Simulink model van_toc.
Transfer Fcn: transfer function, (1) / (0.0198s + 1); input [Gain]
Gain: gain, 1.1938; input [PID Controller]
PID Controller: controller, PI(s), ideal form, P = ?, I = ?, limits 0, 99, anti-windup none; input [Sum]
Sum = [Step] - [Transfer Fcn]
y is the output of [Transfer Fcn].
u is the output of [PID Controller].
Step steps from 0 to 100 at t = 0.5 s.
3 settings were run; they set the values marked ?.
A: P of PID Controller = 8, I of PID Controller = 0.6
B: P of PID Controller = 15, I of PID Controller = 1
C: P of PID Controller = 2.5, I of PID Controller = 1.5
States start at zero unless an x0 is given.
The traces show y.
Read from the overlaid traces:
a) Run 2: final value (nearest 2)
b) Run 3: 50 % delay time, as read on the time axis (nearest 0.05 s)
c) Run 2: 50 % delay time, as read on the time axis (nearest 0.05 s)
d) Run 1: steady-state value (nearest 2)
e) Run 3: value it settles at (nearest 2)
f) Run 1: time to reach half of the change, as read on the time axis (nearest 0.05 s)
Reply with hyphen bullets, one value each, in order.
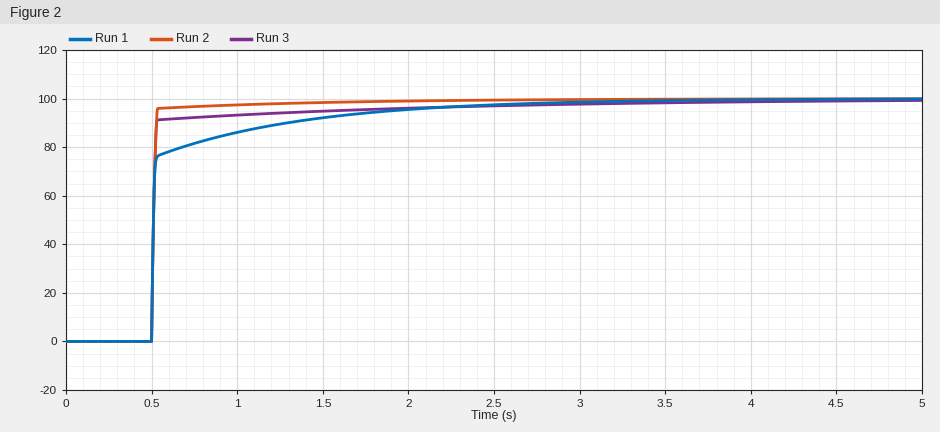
- 100
- 0.50 s
- 0.50 s
- 100
- 100
- 0.50 s
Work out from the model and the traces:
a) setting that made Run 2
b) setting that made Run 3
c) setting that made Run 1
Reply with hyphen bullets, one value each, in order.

- B
- A
- C
